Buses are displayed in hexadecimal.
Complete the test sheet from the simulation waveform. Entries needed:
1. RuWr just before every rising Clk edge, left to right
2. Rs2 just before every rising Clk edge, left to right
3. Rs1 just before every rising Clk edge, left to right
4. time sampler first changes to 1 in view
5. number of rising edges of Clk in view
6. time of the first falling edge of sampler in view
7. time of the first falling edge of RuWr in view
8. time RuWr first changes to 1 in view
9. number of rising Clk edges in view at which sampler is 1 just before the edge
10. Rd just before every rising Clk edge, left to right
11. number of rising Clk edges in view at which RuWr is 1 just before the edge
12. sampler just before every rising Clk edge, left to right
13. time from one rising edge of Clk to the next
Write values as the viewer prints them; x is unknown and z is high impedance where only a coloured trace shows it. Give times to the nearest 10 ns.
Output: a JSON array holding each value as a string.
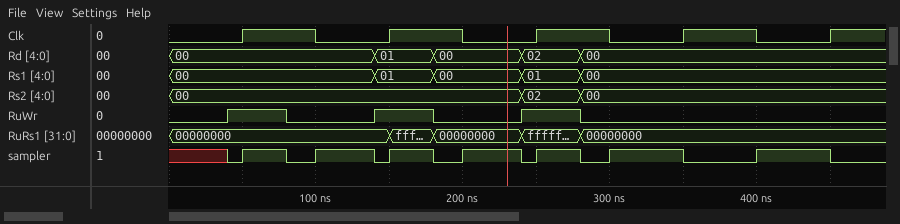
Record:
["1 1 1 0 0", "00, 00, 02, 00, 00", "00, 01, 01, 00, 00", "50 ns", "5", "80 ns", "80 ns", "40 ns", "2", "00, 01, 02, 00, 00", "3", "0 0 0 1 1", "100 ns"]
